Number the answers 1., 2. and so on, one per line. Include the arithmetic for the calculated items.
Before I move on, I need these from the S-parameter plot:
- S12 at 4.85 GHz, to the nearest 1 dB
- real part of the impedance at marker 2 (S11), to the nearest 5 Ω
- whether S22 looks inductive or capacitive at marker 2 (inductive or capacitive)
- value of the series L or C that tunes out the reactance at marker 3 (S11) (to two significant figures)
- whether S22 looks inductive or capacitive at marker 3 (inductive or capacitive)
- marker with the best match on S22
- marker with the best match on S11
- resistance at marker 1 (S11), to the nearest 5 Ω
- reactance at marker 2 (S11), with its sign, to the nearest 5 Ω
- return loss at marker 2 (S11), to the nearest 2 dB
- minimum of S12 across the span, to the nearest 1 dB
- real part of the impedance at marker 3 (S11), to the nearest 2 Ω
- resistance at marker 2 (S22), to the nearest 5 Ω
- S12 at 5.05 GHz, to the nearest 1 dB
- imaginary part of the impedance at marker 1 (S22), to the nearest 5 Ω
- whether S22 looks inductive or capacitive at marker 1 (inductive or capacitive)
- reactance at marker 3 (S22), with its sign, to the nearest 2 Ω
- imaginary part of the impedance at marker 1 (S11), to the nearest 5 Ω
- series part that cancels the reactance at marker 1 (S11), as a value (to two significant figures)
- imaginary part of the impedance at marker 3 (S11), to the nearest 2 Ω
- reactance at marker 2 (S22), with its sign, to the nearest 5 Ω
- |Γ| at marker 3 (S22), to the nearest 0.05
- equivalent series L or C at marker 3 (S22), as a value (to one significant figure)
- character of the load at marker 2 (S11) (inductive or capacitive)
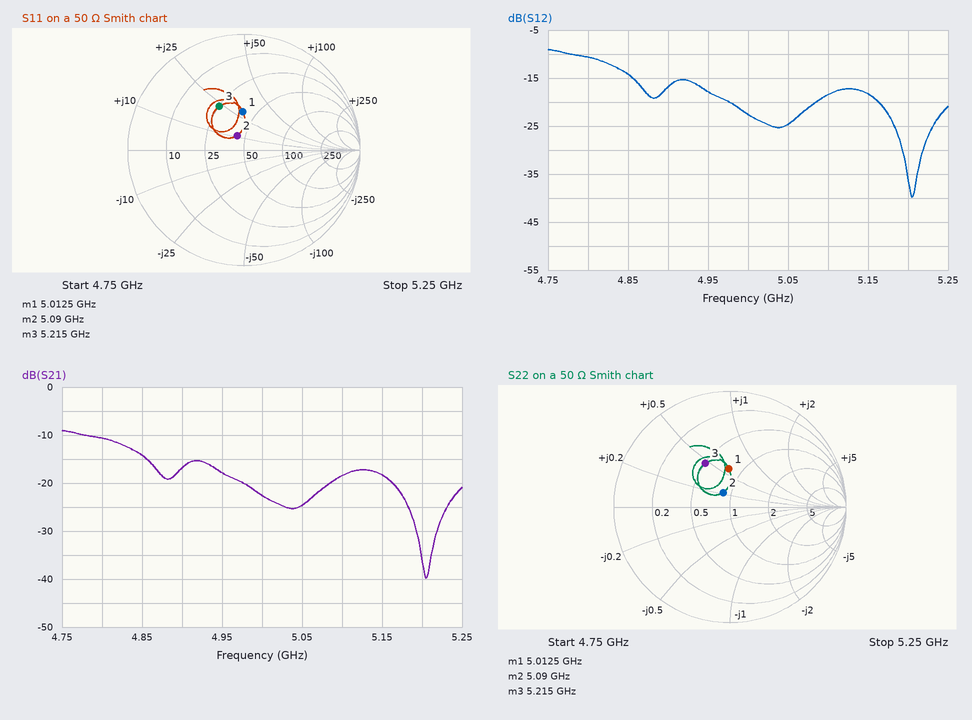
1. -14 dB
2. 45 Ω
3. inductive
4. C = 1/(2π × 5.215 GHz × 24 Ω) ≈ 1.3 pF
5. inductive
6. marker 2
7. marker 2
8. 40 Ω
9. +10 Ω
10. 18 dB
11. -40 dB
12. 26 Ω
13. 45 Ω
14. -25 dB
15. +30 Ω
16. inductive
17. +24 Ω
18. +30 Ω
19. C = 1/(2π × 5.0125 GHz × 30 Ω) ≈ 1.1 pF
20. +24 Ω
21. +10 Ω
22. 0.45
23. L = 24 Ω/(2π × 5.215 GHz) ≈ 732 pH, so 700 pH to one significant figure
24. inductive
